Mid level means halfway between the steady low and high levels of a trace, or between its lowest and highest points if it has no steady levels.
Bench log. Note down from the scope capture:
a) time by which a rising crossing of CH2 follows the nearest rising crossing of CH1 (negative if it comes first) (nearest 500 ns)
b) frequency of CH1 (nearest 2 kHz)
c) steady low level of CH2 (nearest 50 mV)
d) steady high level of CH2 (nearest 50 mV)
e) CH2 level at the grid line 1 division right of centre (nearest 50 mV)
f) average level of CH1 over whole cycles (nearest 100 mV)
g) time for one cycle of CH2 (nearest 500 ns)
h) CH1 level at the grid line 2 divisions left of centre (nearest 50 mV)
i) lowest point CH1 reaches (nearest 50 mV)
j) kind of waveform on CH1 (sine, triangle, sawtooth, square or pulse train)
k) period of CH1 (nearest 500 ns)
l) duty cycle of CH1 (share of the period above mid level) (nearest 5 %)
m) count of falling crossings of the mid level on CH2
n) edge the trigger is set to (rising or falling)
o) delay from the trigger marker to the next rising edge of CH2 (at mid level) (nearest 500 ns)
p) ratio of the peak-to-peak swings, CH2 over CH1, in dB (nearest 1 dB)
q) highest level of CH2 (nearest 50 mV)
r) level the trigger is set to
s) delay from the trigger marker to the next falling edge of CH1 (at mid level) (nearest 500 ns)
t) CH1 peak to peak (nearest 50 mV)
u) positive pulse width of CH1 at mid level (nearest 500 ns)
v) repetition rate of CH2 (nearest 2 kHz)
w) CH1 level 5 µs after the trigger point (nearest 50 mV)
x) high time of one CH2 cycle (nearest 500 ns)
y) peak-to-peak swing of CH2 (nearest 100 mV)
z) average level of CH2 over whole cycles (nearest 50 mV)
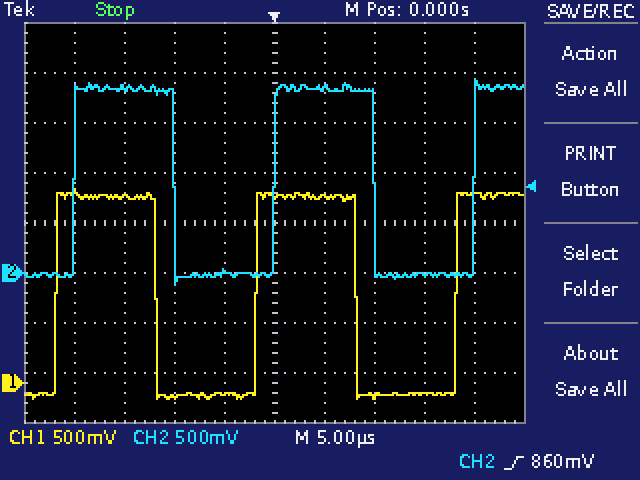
+2.0 µs
50 kHz
0 mV
1.85 V
1.85 V
900 mV
20.0 µs
-150 mV
-150 mV
square
20.0 µs
50 %
2
rising
20.0 µs
0 dB
1.95 V
860 mV
8.0 µs
2.10 V
10.0 µs
50 kHz
1.85 V
10.0 µs
2.10 V
900 mV
